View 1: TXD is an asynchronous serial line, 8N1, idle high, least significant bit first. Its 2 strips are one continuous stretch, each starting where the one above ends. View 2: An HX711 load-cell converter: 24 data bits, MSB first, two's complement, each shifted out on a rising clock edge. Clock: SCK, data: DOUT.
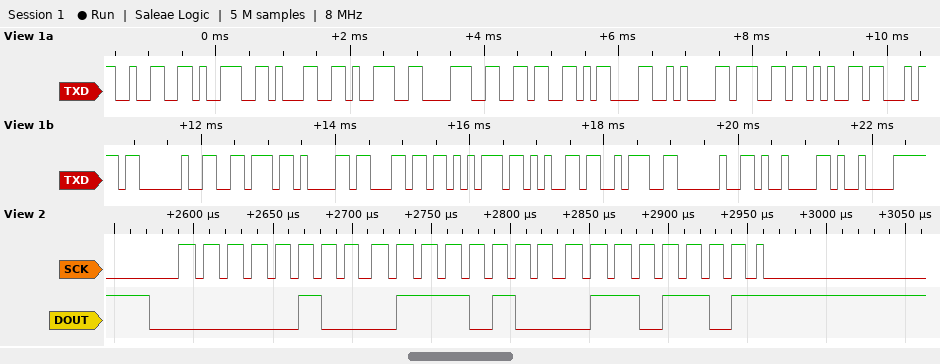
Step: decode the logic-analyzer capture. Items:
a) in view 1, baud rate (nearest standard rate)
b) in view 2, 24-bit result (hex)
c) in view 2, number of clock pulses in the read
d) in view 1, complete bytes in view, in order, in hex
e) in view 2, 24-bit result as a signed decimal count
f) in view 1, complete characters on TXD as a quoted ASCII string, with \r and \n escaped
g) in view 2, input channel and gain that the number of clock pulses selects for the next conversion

9600 baud
0x04746D
25
32 39 31 39 38 36 0D 0A 67 65 74 20 76 61 6C 75 65 3A 20 09 09
291949
"291986\r\nget value: \t\t"
channel A, gain 128
